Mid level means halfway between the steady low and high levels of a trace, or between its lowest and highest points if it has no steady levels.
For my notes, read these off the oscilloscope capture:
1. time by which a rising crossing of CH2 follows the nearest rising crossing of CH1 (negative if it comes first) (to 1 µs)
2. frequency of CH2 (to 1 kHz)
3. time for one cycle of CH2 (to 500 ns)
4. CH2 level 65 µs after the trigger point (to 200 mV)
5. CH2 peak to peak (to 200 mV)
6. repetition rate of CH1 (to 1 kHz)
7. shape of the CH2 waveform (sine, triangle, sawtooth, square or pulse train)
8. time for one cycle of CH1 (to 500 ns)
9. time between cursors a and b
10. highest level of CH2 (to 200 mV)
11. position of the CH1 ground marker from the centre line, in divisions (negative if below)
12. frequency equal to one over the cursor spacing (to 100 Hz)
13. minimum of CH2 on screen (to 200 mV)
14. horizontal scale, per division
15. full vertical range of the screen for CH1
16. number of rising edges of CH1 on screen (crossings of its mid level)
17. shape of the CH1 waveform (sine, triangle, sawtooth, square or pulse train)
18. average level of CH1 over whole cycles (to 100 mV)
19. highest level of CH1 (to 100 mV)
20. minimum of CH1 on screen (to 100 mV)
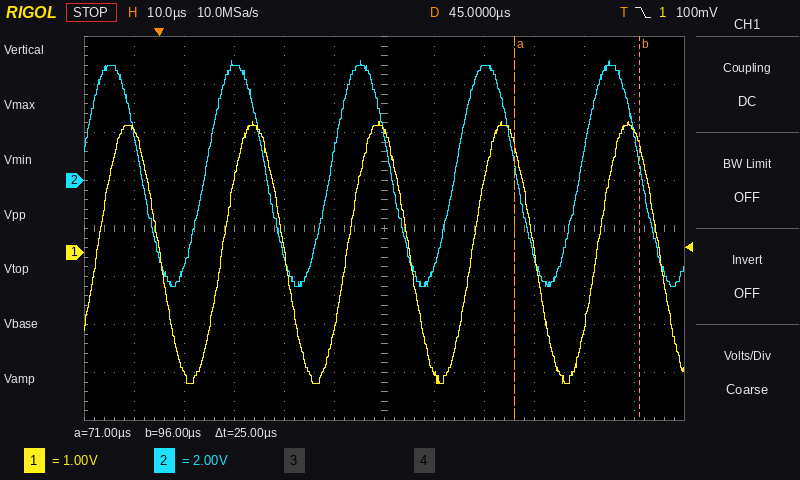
-3 µs
40 kHz
25.0 µs
4.8 V
9.4 V
40 kHz
sine
25.0 µs
25 µs
5.0 V
-0.5 div
40.0 kHz
-4.4 V
10 µs
8 V
5
sine
0.0 V
2.7 V
-2.7 V
